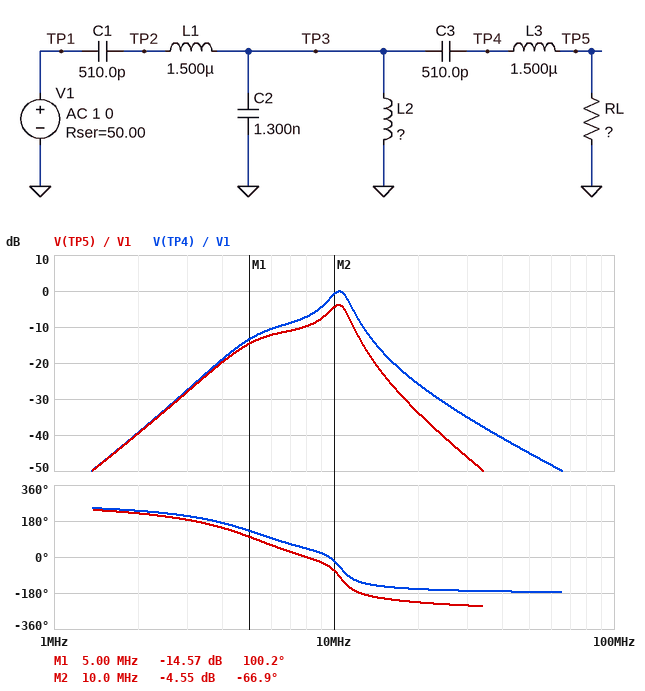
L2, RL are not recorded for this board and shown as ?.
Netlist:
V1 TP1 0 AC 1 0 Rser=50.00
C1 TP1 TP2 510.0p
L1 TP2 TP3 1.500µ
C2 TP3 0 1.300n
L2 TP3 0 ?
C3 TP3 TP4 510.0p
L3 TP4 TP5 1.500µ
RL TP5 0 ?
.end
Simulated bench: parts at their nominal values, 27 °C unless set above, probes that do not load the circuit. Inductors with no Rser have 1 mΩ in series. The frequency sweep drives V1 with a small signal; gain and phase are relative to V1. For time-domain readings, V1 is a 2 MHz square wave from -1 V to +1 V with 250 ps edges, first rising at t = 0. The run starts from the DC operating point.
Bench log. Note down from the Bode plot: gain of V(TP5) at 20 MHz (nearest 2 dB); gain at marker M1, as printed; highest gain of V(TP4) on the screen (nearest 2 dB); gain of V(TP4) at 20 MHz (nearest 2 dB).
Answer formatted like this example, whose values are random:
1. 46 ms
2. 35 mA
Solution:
1. -34 dB
2. -14.57 dB
3. 0 dB
4. -26 dB
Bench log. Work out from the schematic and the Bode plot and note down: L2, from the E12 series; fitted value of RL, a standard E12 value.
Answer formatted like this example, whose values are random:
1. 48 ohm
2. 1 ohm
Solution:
1. 220 nH
2. 82 Ω
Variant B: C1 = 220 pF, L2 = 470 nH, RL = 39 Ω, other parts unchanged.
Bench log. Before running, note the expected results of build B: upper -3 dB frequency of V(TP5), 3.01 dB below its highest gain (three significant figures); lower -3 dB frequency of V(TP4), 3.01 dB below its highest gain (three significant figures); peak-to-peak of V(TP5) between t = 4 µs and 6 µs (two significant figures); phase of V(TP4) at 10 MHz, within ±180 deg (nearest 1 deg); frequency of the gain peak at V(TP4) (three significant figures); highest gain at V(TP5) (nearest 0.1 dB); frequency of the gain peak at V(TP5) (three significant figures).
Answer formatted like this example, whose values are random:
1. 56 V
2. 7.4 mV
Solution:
1. 9.51 MHz
2. 5.75 MHz
3. 450 mV
4. -65 deg
5. 7.67 MHz
6. -7.5 dB
7. 7.10 MHz
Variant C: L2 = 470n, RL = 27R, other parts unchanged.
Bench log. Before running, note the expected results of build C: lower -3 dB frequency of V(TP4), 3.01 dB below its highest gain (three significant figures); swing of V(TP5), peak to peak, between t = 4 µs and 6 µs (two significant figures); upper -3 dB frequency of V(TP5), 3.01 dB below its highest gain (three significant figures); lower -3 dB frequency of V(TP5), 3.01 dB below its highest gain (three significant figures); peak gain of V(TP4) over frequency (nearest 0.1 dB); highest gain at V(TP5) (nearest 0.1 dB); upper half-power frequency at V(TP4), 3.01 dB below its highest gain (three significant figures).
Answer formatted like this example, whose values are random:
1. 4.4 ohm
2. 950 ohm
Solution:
1. 6.23 MHz
2. 380 mV
3. 9.38 MHz
4. 4.03 MHz
5. 1.1 dB
6. -8.7 dB
7. 9.57 MHz
